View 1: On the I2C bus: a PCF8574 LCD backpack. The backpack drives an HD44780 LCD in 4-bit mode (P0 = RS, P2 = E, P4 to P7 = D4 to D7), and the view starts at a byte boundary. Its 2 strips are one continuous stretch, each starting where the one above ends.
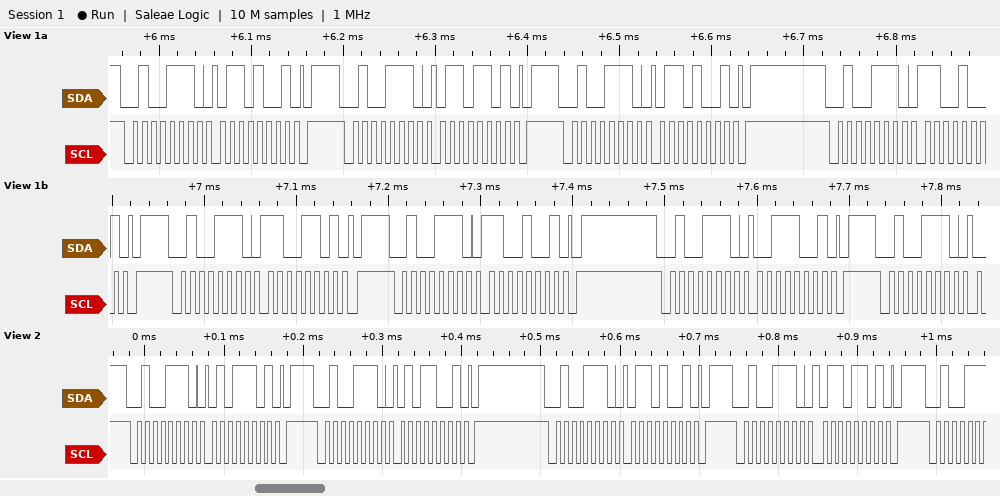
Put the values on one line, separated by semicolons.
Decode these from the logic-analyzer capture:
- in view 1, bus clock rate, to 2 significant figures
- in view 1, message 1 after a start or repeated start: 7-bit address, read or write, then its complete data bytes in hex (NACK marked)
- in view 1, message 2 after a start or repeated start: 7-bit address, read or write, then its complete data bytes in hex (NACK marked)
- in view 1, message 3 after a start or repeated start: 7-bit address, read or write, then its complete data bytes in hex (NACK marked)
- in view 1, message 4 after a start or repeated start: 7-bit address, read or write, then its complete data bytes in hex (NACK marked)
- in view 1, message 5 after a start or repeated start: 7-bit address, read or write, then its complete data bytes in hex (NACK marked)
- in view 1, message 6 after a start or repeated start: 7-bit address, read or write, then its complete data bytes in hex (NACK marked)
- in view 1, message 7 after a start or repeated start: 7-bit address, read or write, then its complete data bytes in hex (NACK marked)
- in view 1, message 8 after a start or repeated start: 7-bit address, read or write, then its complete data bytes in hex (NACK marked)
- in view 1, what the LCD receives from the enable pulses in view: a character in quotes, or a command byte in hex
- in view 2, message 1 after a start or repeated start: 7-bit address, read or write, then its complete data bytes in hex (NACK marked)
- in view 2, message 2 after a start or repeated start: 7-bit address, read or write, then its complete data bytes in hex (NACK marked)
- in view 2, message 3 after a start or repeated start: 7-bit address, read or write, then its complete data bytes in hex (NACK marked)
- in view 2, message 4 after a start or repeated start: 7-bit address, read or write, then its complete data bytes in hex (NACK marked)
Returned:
100 kHz; 0x27 write: 69; 0x27 write: 6D; 0x27 write: 69; 0x27 write: C9; 0x27 write: CD; 0x27 write: C9; 0x27 write: 39; 0x27 write; 'l'; 0x27 write: 5D; 0x27 write: 59; 0x27 write: 69; 0x27 write: 6D
